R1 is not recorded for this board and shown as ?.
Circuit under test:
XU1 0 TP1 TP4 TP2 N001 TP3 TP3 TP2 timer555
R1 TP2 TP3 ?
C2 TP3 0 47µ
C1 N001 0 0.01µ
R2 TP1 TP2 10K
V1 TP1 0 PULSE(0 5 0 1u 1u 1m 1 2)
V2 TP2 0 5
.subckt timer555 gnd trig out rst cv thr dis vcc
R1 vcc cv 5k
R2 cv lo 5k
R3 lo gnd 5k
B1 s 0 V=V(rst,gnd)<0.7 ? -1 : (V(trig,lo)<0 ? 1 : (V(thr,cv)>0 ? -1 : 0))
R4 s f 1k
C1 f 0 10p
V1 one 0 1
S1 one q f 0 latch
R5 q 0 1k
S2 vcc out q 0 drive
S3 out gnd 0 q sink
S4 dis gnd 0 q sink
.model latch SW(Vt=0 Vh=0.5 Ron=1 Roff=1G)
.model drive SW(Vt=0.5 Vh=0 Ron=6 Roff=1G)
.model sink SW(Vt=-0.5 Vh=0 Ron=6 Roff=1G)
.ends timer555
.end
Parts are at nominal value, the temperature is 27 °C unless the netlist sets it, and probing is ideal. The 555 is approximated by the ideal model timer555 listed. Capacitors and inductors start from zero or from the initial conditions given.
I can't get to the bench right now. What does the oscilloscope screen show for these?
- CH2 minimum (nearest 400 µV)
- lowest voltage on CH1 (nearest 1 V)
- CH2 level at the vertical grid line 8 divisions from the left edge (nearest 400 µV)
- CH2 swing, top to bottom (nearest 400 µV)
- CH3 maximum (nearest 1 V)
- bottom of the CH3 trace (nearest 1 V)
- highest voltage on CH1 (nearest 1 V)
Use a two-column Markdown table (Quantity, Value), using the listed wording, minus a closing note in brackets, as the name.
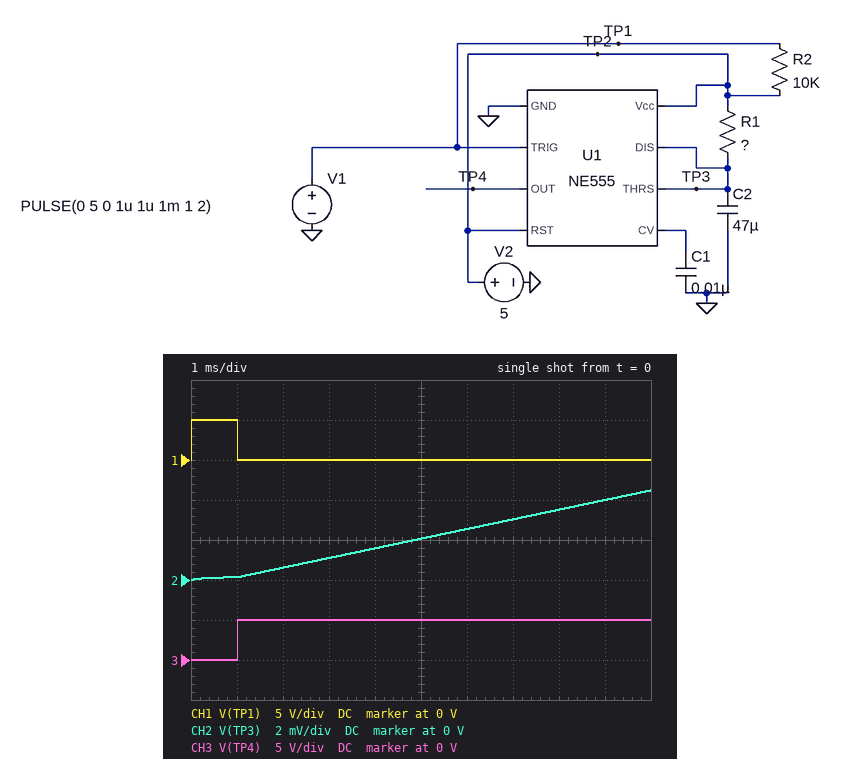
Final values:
| Quantity | Value |
|---|---|
| CH2 minimum | 0 V |
| lowest voltage on CH1 | 0 V |
| CH2 level at the vertical grid line 8 divisions from the left edge | 3.6 mV |
| CH2 swing, top to bottom | 4.4 mV |
| CH3 maximum | 5 V |
| bottom of the CH3 trace | 0 V |
| highest voltage on CH1 | 5 V |
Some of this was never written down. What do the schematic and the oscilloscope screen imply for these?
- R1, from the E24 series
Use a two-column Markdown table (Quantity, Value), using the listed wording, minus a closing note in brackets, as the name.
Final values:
| Quantity | Value |
|---|---|
| R1, from the E24 series | 220 kΩ |
